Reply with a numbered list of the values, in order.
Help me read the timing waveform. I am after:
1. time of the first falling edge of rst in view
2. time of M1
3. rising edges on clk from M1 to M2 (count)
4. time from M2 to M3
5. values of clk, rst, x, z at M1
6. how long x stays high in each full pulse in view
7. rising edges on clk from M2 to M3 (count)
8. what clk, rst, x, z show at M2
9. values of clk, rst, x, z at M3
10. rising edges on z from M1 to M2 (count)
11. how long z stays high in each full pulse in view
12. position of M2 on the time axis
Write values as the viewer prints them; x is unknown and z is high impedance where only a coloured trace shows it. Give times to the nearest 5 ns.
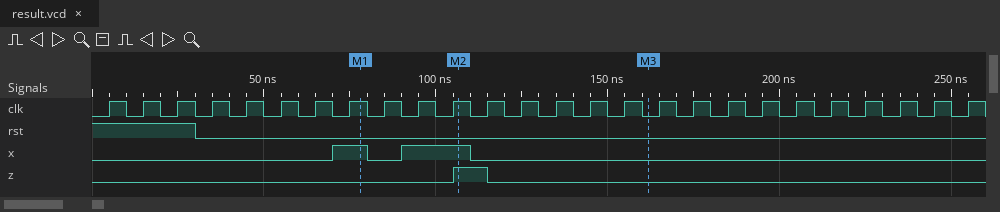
1. 30 ns
2. 80 ns
3. 3
4. 55 ns
5. clk=1, rst=0, x=1, z=0
6. 10 ns, 20 ns
7. 5
8. clk=1, rst=0, x=1, z=1
9. clk=0, rst=0, x=0, z=0
10. 1
11. 10 ns
12. 105 ns
